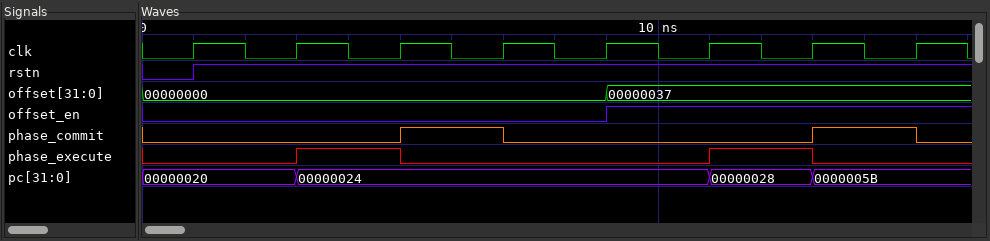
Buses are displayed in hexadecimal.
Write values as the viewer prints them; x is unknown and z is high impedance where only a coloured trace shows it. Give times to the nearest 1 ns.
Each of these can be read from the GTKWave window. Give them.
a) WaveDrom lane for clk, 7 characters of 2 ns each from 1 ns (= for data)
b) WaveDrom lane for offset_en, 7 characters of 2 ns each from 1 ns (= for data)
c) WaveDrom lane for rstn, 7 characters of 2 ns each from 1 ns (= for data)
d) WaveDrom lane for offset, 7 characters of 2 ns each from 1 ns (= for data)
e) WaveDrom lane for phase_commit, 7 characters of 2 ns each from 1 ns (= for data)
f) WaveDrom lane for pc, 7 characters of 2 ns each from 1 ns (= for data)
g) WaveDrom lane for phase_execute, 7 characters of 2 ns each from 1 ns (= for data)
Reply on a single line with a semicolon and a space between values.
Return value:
{name: 'clk', wave: 'p......'}; {name: 'offset_en', wave: '0...1..'}; {name: 'rstn', wave: '1......'}; {name: 'offset', wave: '=...=..', data: '00000000 00000037'}; {name: 'phase_commit', wave: '0.10..1'}; {name: 'pc', wave: '==...==', data: '00000020 00000024 00000028 0000005B'}; {name: 'phase_execute', wave: '010..10'}
